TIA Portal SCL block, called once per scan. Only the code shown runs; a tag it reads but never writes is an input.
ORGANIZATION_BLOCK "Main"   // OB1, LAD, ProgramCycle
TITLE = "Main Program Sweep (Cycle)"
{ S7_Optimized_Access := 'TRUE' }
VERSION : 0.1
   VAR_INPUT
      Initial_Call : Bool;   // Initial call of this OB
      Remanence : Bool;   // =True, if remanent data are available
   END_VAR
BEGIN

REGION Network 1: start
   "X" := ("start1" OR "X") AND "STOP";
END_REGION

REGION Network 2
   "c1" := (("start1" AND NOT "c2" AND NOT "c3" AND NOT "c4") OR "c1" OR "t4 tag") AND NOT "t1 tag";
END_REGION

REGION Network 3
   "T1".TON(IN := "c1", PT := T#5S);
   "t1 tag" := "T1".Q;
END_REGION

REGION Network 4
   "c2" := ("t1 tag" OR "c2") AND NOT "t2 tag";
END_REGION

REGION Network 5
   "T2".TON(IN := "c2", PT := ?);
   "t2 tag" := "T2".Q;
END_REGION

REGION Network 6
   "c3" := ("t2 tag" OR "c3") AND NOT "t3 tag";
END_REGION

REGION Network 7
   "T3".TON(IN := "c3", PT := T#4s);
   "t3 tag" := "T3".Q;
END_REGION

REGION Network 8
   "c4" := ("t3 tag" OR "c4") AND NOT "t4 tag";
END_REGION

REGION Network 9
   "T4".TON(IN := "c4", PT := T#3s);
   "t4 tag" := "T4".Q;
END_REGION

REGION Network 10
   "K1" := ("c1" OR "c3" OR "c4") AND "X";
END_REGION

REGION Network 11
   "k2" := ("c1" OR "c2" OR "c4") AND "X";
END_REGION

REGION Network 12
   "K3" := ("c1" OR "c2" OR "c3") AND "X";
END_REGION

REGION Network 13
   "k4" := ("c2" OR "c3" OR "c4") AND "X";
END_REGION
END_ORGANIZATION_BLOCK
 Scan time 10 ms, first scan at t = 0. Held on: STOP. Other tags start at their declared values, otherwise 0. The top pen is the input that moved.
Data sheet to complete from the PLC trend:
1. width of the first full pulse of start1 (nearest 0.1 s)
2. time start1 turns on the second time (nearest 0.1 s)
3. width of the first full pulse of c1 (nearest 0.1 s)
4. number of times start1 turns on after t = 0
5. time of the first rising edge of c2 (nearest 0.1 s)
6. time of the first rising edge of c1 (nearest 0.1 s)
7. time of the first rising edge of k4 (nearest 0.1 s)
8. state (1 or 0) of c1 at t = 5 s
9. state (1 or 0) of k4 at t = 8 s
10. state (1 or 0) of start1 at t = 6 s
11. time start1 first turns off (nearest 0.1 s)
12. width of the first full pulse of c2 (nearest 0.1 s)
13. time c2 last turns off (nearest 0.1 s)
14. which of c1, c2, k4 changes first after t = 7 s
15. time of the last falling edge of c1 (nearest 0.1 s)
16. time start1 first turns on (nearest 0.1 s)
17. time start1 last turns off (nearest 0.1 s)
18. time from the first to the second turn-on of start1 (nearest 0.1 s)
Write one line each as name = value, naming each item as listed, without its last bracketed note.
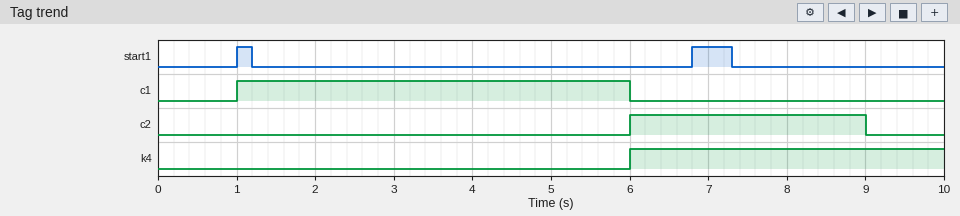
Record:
width of the first full pulse of start1 = 0.2 s
time start1 turns on the second time = 6.8 s
width of the first full pulse of c1 = 5.0 s
number of times start1 turns on after t = 0 = 2
time of the first rising edge of c2 = 6.0 s
time of the first rising edge of c1 = 1.0 s
time of the first rising edge of k4 = 6.0 s
state (1 or 0) of c1 at t = 5 s = 1
state (1 or 0) of k4 at t = 8 s = 1
state (1 or 0) of start1 at t = 6 s = 0
time start1 first turns off = 1.2 s
width of the first full pulse of c2 = 3.0 s
time c2 last turns off = 9.0 s
which of c1, c2, k4 changes first after t = 7 s = c2
time of the last falling edge of c1 = 6.0 s
time start1 first turns on = 1.0 s
time start1 last turns off = 7.3 s
time from the first to the second turn-on of start1 = 5.8 s
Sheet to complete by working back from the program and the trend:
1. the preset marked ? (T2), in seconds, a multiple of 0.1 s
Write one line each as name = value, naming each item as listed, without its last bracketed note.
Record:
the preset marked ? (T2), in seconds, a multiple of 0.1 s = 3.0 s
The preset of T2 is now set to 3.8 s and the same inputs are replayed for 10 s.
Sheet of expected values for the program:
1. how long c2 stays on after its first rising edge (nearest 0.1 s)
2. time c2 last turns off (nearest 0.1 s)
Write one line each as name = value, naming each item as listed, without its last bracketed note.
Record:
how long c2 stays on after its first rising edge = 3.8 s
time c2 last turns off = 9.8 s
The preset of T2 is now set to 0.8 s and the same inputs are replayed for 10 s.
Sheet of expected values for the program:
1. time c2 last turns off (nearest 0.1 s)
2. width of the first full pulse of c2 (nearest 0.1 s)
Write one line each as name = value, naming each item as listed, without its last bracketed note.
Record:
time c2 last turns off = 6.8 s
width of the first full pulse of c2 = 0.8 s
